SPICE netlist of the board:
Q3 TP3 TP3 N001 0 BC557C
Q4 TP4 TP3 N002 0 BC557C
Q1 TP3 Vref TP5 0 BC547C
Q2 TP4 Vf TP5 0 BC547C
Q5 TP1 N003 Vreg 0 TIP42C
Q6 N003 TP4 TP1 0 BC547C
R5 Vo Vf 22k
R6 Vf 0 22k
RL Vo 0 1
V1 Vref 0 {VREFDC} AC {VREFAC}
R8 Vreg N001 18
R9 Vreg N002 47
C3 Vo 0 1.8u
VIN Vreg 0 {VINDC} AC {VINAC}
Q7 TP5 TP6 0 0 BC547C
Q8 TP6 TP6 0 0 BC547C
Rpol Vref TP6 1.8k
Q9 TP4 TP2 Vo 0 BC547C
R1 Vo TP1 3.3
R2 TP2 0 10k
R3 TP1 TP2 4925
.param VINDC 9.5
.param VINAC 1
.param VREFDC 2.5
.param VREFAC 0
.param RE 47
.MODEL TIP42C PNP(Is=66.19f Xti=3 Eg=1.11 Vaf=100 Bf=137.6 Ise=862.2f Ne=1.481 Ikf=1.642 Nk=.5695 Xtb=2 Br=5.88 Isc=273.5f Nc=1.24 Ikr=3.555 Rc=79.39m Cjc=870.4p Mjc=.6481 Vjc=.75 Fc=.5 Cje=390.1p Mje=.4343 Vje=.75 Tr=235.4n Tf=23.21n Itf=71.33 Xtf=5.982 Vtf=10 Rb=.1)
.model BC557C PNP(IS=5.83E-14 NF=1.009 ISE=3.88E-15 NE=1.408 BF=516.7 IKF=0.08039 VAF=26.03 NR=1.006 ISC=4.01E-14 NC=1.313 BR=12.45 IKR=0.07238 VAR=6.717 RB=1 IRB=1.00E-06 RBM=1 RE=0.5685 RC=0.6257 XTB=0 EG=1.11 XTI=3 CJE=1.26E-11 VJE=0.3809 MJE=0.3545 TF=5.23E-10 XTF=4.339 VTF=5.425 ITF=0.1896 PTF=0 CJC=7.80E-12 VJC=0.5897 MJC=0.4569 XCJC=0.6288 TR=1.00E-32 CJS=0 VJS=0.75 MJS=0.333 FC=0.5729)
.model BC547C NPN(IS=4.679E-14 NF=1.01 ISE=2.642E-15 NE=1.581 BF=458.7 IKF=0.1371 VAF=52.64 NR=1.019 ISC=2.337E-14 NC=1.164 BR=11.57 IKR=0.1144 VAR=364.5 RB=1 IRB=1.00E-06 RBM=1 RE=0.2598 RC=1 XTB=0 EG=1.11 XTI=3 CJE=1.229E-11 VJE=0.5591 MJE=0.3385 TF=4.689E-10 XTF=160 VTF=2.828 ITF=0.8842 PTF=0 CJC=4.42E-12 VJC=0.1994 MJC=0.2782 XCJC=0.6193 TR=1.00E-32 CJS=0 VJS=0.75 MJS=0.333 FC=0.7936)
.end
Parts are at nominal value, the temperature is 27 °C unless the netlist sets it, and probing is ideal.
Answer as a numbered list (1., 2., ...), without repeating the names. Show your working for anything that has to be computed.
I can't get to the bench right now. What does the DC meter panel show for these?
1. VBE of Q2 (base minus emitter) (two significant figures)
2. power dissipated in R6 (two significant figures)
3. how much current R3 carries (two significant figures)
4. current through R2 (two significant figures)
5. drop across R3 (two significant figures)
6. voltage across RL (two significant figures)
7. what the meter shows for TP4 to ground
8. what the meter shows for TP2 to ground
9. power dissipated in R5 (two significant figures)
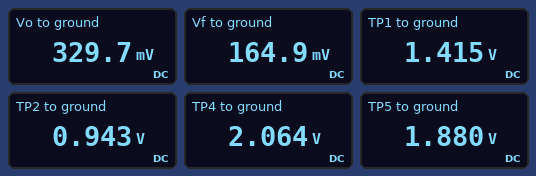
1. 164.9 mV - 1.88 V = -1.7 V
2. (164.9 mV)^2 / 22 kΩ = 1.2 µW
3. (1.415 V - 943 mV) / 4.925 kΩ = 96 µA
4. (943 mV) / 10 kΩ = 94 µA
5. 1.415 V - 943 mV = 470 mV
6. 329.7 mV = 330 mV
7. 2.064 V
8. 0.943 V
9. (329.7 mV - 164.9 mV)^2 / 22 kΩ = 1.2 µW
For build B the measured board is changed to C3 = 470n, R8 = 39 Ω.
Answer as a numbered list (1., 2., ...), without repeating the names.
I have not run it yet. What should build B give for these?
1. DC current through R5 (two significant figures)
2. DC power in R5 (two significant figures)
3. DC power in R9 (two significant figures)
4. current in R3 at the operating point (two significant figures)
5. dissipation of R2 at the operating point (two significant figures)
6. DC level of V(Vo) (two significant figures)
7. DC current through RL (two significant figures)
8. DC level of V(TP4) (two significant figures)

1. 7.6 µA
2. 1.3 µW
3. 50 µW
4. 98 µA
5. 92 µW
6. 340 mV
7. 340 mA
8. 2.1 V
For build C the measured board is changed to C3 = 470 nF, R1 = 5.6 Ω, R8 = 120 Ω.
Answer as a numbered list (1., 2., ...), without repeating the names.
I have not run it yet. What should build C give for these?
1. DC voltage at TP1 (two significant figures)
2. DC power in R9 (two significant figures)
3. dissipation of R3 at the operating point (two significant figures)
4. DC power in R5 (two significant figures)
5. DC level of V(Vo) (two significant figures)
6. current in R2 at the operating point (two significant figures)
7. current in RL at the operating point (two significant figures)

1. 1.3 V
2. 260 µW
3. 39 µW
4. 440 nW
5. 200 mV
6. 84 µA
7. 200 mA
